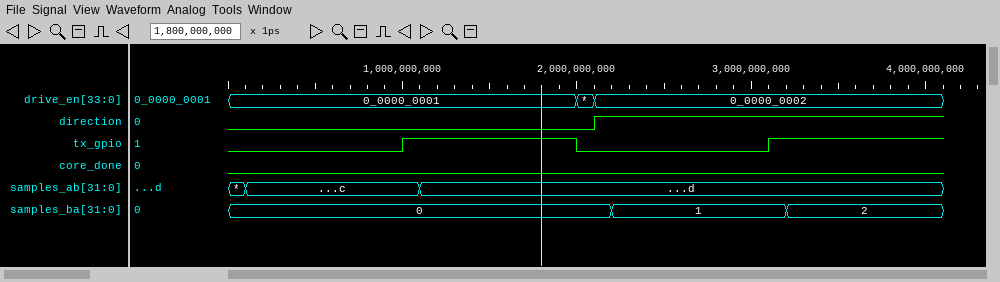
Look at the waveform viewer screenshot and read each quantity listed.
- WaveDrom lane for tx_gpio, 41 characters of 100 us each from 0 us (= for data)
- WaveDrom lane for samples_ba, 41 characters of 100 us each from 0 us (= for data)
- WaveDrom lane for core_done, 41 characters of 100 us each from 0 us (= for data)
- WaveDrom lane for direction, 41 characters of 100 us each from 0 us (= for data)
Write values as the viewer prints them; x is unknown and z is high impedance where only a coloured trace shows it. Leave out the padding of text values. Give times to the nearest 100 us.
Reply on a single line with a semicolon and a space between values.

{name: 'tx_gpio', wave: '0.........1.........0..........1.........'}; {name: 'samples_ba', wave: '=.....................=.........=........', data: '0 1 2'}; {name: 'core_done', wave: '0........................................'}; {name: 'direction', wave: '0....................1...................'}
